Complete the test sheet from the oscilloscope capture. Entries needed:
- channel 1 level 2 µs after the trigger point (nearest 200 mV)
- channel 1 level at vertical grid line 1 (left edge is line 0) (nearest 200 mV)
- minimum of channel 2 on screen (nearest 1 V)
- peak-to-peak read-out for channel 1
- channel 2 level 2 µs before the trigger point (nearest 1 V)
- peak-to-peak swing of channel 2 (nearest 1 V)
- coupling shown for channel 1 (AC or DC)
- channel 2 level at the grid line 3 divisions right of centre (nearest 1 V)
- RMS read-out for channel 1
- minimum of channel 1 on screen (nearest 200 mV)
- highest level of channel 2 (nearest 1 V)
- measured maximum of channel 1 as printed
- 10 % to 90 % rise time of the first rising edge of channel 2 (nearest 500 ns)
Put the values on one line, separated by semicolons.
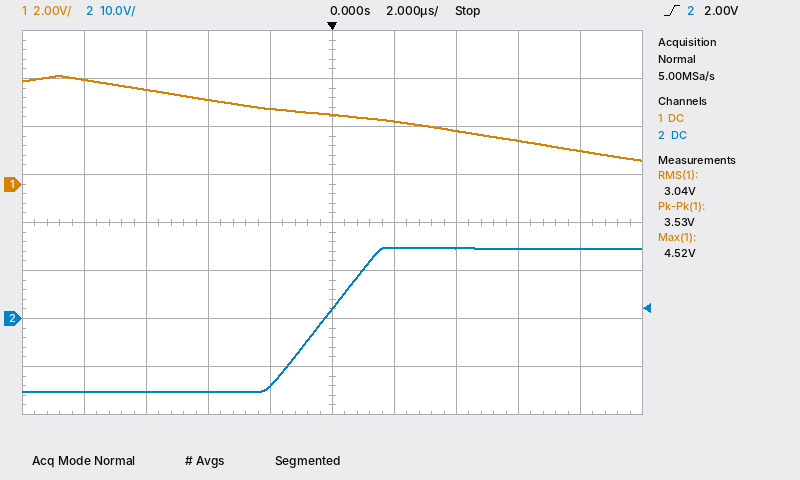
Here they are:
2.6 V; 4.4 V; -15 V; 3.53 V; -14 V; 30 V; DC; 15 V; 3.04 V; 1.0 V; 15 V; 4.52 V; 3.0 µs
